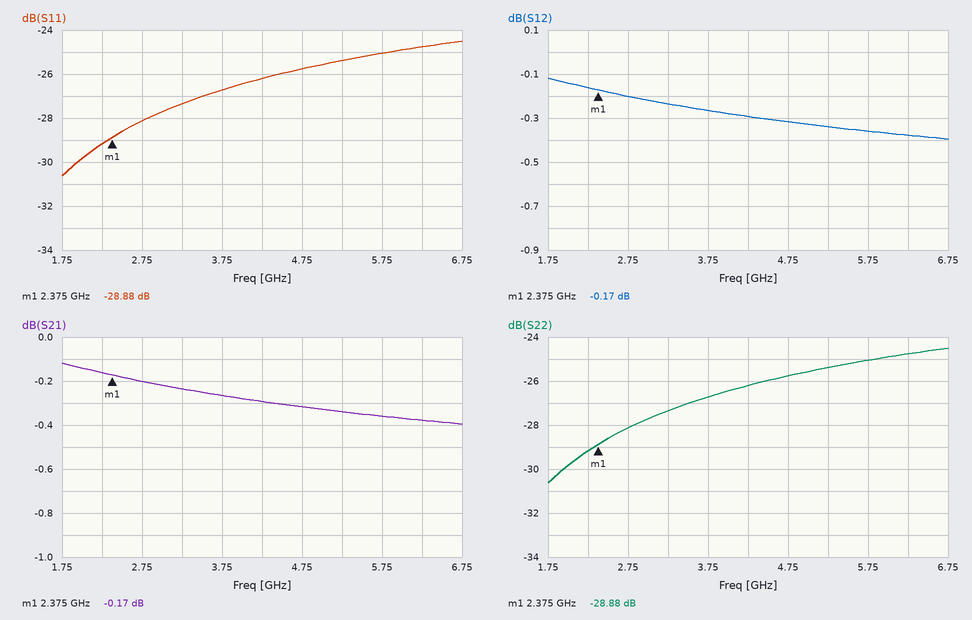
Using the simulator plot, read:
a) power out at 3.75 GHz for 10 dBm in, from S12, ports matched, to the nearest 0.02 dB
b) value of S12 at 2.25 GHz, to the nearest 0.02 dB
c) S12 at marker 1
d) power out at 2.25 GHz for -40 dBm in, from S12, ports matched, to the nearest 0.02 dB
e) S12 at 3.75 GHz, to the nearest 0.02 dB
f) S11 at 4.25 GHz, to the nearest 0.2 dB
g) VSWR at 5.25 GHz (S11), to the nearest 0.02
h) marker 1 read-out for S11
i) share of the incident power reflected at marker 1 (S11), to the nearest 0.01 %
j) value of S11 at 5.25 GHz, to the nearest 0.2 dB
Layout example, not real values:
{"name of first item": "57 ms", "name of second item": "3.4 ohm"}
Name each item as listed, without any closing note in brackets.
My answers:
{"power out at 3.75 GHz for 10 dBm in, from S12, ports matched, to the nearest 0.02 dB": "9.74 dBm", "value of S12 at 2.25 GHz, to the nearest 0.02 dB": "-0.16 dB", "S12 at marker 1": "-0.17 dB", "power out at 2.25 GHz for -40 dBm in, from S12, ports matched, to the nearest 0.02 dB": "-40.16 dBm", "S12 at 3.75 GHz, to the nearest 0.02 dB": "-0.26 dB", "S11 at 4.25 GHz, to the nearest 0.2 dB": "-26.2 dB", "VSWR at 5.25 GHz (S11), to the nearest 0.02": "1.12", "marker 1 read-out for S11": "-28.88 dB", "share of the incident power reflected at marker 1 (S11), to the nearest 0.01 %": "0.13 %", "value of S11 at 5.25 GHz, to the nearest 0.2 dB": "-25.4 dB"}
